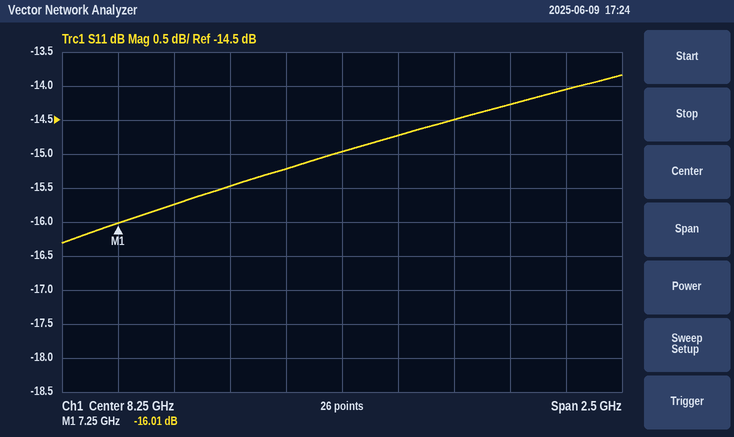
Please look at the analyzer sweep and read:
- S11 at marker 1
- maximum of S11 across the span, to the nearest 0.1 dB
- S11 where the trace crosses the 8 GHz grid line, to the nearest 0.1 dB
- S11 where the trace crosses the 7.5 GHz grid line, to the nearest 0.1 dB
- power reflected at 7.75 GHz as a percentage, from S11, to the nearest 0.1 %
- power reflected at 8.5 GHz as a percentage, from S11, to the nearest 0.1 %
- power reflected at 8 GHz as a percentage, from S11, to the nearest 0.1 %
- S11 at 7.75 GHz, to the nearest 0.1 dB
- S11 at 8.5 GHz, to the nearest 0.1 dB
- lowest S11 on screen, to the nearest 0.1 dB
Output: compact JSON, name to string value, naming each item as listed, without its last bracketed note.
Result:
{"S11 at marker 1": "-16.01 dB", "maximum of S11 across the span, to the nearest 0.1 dB": "-13.8 dB", "S11 where the trace crosses the 8 GHz grid line, to the nearest 0.1 dB": "-15.2 dB", "S11 where the trace crosses the 7.5 GHz grid line, to the nearest 0.1 dB": "-15.7 dB", "power reflected at 7.75 GHz as a percentage, from S11, to the nearest 0.1 %": "2.8 %", "power reflected at 8.5 GHz as a percentage, from S11, to the nearest 0.1 %": "3.4 %", "power reflected at 8 GHz as a percentage, from S11, to the nearest 0.1 %": "3.0 %", "S11 at 7.75 GHz, to the nearest 0.1 dB": "-15.5 dB", "S11 at 8.5 GHz, to the nearest 0.1 dB": "-14.7 dB", "lowest S11 on screen, to the nearest 0.1 dB": "-16.3 dB"}
